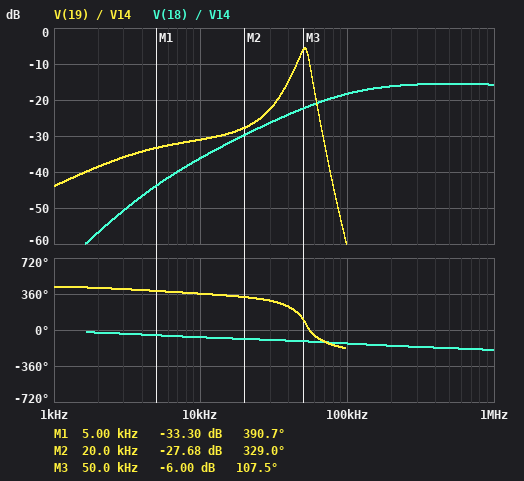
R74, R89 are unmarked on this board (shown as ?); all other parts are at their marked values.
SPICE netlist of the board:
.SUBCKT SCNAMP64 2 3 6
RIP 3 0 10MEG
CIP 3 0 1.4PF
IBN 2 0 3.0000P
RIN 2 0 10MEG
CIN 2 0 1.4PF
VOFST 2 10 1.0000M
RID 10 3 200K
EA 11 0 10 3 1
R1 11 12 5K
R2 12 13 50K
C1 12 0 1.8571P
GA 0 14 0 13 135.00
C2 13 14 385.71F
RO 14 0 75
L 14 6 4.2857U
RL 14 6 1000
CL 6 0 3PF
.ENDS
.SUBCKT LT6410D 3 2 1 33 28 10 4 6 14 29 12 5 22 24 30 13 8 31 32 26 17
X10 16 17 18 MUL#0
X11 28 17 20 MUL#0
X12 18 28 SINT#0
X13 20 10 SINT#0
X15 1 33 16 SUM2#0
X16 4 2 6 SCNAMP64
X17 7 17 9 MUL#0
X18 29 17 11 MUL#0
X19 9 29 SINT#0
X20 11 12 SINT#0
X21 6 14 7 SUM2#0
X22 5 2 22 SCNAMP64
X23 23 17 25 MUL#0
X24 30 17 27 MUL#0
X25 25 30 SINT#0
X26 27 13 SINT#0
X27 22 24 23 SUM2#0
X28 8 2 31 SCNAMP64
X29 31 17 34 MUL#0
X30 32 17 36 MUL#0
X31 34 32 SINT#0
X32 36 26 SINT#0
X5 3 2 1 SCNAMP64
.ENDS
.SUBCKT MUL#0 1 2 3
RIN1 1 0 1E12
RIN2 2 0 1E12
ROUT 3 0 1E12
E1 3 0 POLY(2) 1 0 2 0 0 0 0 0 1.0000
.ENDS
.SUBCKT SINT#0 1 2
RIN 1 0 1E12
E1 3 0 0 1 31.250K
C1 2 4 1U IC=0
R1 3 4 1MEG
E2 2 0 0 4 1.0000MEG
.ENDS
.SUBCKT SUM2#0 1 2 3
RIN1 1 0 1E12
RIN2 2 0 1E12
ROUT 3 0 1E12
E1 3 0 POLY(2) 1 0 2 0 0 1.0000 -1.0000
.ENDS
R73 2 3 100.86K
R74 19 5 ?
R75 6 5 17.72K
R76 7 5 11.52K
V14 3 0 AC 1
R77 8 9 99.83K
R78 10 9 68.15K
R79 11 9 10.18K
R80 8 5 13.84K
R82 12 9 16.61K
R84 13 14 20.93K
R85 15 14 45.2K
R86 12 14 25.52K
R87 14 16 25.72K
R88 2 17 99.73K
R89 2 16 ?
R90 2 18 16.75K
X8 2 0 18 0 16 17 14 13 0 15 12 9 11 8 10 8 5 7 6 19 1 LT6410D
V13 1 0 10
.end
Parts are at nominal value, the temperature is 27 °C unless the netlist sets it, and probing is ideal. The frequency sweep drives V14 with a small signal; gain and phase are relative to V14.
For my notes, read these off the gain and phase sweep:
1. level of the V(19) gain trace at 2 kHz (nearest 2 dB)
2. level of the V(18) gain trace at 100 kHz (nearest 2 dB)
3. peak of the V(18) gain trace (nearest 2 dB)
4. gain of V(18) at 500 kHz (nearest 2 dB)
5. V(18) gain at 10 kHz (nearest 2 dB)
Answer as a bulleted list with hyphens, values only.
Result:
- -38 dB
- -18 dB
- -16 dB
- -16 dB
- -36 dB
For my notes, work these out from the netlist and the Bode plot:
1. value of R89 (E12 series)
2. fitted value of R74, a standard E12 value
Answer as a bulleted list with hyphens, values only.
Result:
- 8.2 kΩ
- 8.2 kΩ
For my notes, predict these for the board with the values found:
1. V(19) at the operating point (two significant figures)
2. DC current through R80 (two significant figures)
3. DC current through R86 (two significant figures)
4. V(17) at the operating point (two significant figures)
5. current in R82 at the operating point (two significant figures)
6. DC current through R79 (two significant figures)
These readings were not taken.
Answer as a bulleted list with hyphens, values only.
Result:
- 3.0 mV
- 100 nA
- 110 nA
- 20 mV
- 170 nA
- 140 nA
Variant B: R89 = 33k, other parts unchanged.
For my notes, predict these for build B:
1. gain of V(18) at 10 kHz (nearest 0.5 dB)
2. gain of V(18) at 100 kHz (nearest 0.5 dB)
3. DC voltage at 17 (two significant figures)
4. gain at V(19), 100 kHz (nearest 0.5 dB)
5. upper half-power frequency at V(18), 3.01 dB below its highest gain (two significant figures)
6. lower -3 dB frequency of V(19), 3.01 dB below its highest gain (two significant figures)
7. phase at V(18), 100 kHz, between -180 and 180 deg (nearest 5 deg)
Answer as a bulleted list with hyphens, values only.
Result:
- -27.5 dB
- -15.5 dB
- 11 mV
- -58.0 dB
- 6.4 MHz
- 46 kHz
- -165 deg
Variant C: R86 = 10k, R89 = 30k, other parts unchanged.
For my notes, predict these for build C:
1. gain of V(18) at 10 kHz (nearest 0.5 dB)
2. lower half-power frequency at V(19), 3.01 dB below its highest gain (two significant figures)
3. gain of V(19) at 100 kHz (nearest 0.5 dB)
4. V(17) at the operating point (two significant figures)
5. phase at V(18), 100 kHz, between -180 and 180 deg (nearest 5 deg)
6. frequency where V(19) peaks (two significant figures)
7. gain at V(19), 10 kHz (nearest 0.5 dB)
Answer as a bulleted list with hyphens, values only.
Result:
- -28.0 dB
- 49 kHz
- -54.0 dB
- 11 mV
- -165 deg
- 52 kHz
- -31.5 dB
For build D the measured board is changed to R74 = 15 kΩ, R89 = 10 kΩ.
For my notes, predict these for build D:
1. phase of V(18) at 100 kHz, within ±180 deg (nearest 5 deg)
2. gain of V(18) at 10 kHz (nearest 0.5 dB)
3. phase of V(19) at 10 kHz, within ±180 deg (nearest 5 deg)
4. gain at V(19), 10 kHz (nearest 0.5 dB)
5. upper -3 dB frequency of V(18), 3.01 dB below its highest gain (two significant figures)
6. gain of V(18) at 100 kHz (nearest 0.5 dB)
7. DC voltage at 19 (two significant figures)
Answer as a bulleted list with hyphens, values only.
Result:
- -140 deg
- -34.5 dB
- 0 deg
- -24.0 dB
- 3.3 MHz
- -17.5 dB
- 4.7 mV
